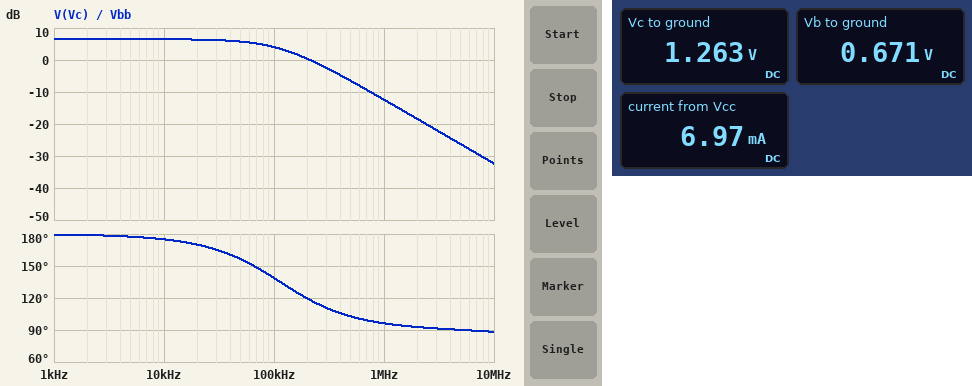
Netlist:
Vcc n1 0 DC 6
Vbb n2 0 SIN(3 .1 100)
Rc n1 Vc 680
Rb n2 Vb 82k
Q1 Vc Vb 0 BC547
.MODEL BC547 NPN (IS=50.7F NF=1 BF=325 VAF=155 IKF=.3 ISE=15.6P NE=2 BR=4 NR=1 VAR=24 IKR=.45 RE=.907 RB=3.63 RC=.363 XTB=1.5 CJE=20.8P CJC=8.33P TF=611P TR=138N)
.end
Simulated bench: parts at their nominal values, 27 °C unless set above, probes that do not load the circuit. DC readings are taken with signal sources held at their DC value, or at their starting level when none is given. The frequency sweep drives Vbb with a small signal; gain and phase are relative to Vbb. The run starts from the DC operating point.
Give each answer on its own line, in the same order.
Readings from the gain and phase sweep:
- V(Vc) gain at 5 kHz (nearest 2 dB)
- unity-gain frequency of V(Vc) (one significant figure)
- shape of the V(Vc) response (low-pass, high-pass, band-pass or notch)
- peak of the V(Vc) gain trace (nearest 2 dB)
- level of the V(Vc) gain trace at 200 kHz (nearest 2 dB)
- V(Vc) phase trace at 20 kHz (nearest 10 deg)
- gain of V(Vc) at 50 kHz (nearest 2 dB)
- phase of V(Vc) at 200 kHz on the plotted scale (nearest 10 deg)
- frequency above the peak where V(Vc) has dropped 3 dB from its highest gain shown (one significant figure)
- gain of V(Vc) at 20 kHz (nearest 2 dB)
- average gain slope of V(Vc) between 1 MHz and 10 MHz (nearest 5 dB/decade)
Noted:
6 dB
200 kHz
low-pass
6 dB
0 dB
170 deg
6 dB
120 deg
100 kHz
6 dB
-20 dB/decade
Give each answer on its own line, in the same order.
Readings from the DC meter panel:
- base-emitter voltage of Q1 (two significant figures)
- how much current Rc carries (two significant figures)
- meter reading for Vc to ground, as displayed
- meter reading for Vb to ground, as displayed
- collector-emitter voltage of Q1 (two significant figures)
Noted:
670 mV
7.0 mA
1.263 V
0.671 V
1.3 V
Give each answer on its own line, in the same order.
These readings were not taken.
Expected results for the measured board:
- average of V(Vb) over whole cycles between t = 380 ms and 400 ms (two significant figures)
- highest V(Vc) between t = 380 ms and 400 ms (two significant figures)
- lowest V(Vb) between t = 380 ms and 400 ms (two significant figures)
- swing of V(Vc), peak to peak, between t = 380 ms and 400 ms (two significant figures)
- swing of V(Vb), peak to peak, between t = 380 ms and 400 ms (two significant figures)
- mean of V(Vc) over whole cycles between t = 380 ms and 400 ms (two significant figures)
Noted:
670 mV
1.5 V
670 mV
420 mV
3.0 mV
1.3 V
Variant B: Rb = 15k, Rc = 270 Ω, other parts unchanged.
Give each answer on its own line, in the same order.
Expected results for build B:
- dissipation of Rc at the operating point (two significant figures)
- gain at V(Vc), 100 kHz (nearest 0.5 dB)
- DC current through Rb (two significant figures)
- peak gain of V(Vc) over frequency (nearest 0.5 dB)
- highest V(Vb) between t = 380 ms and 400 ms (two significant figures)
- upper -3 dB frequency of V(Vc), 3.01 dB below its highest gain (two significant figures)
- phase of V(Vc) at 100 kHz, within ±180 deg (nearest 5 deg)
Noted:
130 mW
-32.5 dB
150 µA
-32.0 dB
720 mV
290 kHz
160 deg
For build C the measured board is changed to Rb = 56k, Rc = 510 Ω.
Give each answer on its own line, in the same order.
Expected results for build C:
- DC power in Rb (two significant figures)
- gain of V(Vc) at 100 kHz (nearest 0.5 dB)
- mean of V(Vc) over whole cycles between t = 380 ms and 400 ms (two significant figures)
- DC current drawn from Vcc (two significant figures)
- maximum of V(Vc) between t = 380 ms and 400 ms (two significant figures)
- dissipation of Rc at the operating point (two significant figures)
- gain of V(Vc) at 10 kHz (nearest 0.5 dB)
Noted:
96 µW
5.0 dB
700 mV
10 mA
930 mV
55 mW
7.0 dB
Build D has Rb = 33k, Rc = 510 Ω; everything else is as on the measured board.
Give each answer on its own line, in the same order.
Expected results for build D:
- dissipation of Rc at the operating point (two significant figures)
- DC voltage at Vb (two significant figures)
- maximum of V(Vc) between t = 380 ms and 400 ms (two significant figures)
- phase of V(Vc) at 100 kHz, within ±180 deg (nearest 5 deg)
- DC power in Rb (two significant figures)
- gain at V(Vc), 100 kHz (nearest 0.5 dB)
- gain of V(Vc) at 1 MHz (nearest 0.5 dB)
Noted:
67 mW
690 mV
140 mV
160 deg
160 µW
-30.5 dB
-41.5 dB
